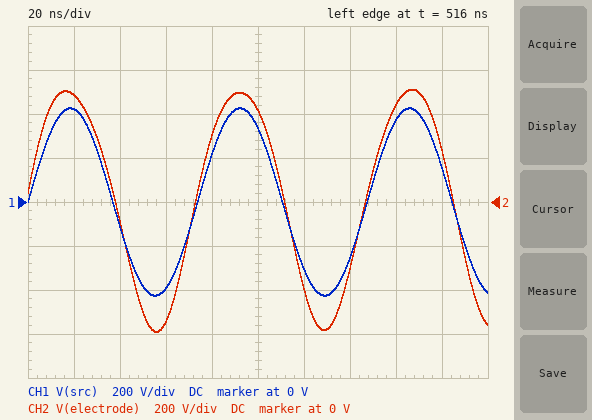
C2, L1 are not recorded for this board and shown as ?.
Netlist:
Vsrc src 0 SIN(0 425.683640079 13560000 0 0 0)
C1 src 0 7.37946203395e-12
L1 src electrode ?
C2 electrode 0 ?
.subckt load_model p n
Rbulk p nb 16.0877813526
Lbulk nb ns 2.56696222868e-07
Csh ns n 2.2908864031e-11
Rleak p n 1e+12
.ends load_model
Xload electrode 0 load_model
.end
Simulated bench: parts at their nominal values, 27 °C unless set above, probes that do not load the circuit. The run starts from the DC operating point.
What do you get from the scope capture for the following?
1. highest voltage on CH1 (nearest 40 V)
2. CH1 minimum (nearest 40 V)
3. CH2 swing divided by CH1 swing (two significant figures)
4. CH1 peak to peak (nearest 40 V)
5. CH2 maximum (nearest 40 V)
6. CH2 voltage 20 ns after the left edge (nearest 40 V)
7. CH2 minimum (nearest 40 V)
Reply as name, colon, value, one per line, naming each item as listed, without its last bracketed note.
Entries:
highest voltage on CH1: 440 V
CH1 minimum: -440 V
CH2 swing divided by CH1 swing: 1.3
CH1 peak to peak: 840 V
CH2 maximum: 520 V
CH2 voltage 20 ns after the left edge: 480 V
CH2 minimum: -600 V
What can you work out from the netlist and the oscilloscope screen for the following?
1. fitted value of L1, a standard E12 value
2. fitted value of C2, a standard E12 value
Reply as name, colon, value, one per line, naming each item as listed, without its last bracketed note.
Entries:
fitted value of L1, a standard E12 value: 470 nH
fitted value of C2, a standard E12 value: 39 pF
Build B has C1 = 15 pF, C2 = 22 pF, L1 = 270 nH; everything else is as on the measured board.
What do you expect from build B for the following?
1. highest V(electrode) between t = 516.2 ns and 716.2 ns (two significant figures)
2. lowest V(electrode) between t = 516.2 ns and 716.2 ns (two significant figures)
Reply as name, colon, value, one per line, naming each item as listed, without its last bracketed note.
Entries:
highest V(electrode) between t = 516.2 ns and 716.2 ns: 470 V
lowest V(electrode) between t = 516.2 ns and 716.2 ns: -470 V
